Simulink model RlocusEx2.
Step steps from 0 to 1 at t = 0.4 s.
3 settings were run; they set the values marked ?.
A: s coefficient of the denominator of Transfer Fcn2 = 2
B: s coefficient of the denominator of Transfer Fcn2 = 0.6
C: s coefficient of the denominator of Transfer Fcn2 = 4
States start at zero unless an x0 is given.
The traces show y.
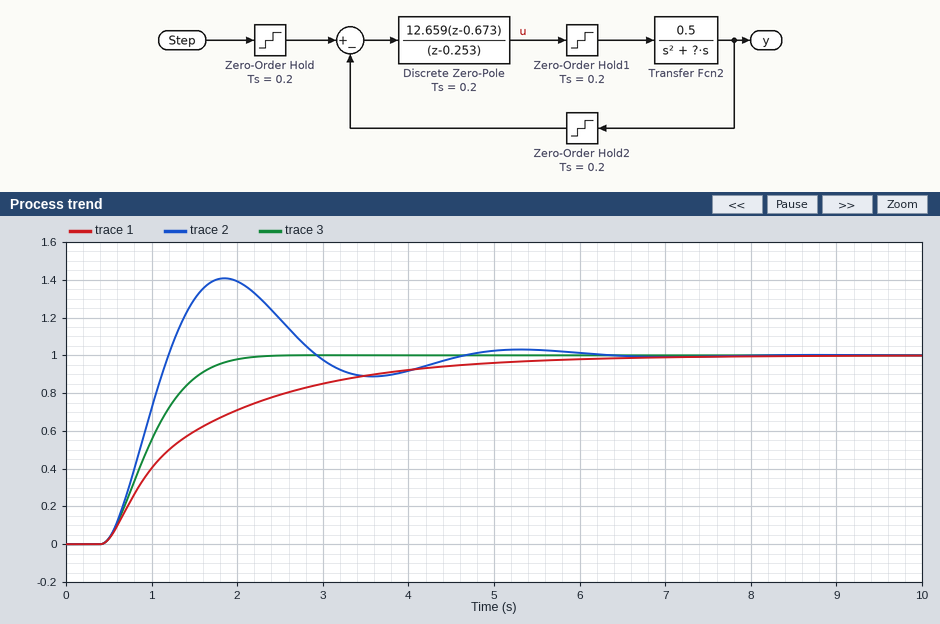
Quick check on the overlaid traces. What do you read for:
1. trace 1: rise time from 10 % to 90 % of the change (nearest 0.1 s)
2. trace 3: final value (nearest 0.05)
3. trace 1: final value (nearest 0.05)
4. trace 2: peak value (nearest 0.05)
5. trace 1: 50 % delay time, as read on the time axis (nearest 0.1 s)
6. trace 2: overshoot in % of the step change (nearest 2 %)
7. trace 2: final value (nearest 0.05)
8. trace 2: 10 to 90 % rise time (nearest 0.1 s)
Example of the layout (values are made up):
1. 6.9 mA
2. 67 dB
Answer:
1. 3.0 s
2. 1.00
3. 1.00
4. 1.40
5. 1.2 s
6. 40 %
7. 1.00
8. 0.5 s
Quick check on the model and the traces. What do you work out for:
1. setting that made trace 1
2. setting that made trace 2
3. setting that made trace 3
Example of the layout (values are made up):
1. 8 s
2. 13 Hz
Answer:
1. C
2. B
3. A
